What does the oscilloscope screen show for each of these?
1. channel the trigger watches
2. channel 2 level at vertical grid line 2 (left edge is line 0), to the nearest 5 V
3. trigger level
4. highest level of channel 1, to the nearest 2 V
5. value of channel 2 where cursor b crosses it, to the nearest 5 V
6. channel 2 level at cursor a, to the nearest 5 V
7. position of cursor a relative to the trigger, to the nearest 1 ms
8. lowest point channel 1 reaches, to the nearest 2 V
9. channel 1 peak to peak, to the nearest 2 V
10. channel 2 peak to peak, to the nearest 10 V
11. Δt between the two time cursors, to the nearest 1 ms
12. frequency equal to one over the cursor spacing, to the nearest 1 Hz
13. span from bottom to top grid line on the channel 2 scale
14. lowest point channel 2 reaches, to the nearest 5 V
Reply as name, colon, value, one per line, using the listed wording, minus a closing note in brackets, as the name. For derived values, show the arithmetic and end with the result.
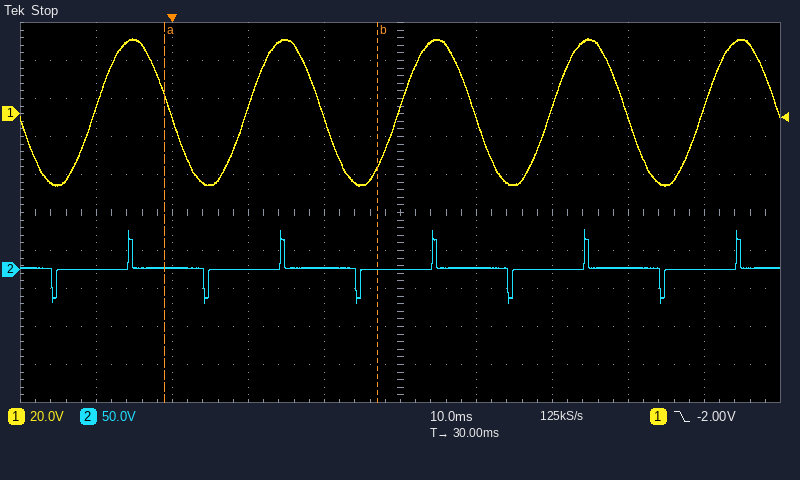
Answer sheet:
channel the trigger watches: channel 1
channel 2 level at vertical grid line 2 (left edge is line 0), to the nearest 5 V: 0 V
trigger level: -2.00 V
highest level of channel 1, to the nearest 2 V: 40 V
value of channel 2 where cursor b crosses it, to the nearest 5 V: 0 V
channel 2 level at cursor a, to the nearest 5 V: 0 V
position of cursor a relative to the trigger, to the nearest 1 ms: -1 ms
lowest point channel 1 reaches, to the nearest 2 V: -38 V
channel 1 peak to peak, to the nearest 2 V: 40 V − (-38 V) = 78 V
channel 2 peak to peak, to the nearest 10 V: 100 V
Δt between the two time cursors, to the nearest 1 ms: 28 ms
frequency equal to one over the cursor spacing, to the nearest 1 Hz: 1 / 28 ms ≈ 36 Hz
span from bottom to top grid line on the channel 2 scale: 500 V
lowest point channel 2 reaches, to the nearest 5 V: -45 V
